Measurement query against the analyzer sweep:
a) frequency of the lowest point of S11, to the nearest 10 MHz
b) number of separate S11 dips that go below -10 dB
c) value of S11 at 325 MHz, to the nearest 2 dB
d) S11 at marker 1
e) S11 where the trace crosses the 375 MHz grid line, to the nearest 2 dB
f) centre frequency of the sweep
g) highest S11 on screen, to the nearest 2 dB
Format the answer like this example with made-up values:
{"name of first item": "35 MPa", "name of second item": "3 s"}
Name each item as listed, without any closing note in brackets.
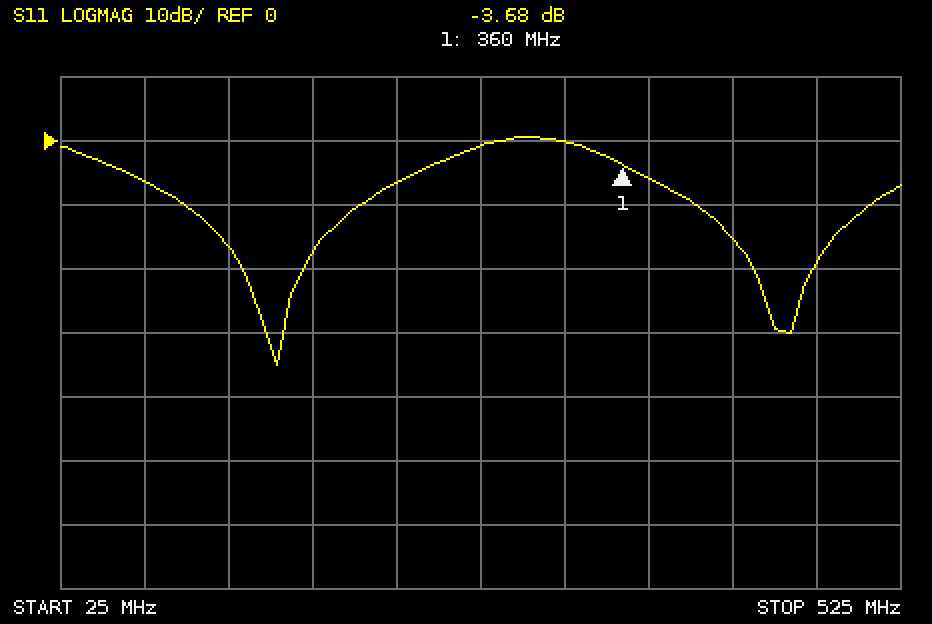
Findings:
{"frequency of the lowest point of S11, to the nearest 10 MHz": "150 MHz", "number of separate S11 dips that go below -10 dB": "2", "value of S11 at 325 MHz, to the nearest 2 dB": "0 dB", "S11 at marker 1": "-3.68 dB", "S11 where the trace crosses the 375 MHz grid line, to the nearest 2 dB": "-6 dB", "centre frequency of the sweep": "275 MHz", "highest S11 on screen, to the nearest 2 dB": "0 dB"}
